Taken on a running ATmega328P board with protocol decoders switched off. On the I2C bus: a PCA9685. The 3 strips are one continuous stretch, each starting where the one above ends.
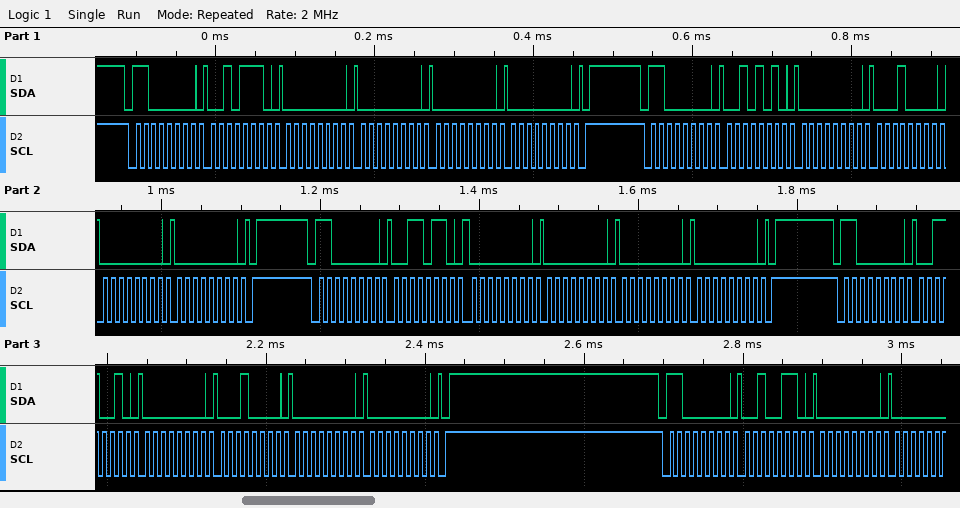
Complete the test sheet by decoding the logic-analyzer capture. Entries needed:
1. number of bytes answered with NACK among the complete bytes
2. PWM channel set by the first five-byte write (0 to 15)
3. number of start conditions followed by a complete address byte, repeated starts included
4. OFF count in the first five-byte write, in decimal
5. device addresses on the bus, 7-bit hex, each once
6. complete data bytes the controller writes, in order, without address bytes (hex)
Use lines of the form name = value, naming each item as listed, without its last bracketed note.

number of bytes answered with NACK among the complete bytes = 0
PWM channel set by the first five-byte write = 10
number of start conditions followed by a complete address byte, repeated starts included = 5
OFF count in the first five-byte write, in decimal = 0
device addresses on the bus, 7-bit hex, each once = 0x60
complete data bytes the controller writes, in order, without address bytes = 2E 00 00 00 00 2A 00 10 00 00 36 00 00 00 00 32 00 10 00 00 26 00
